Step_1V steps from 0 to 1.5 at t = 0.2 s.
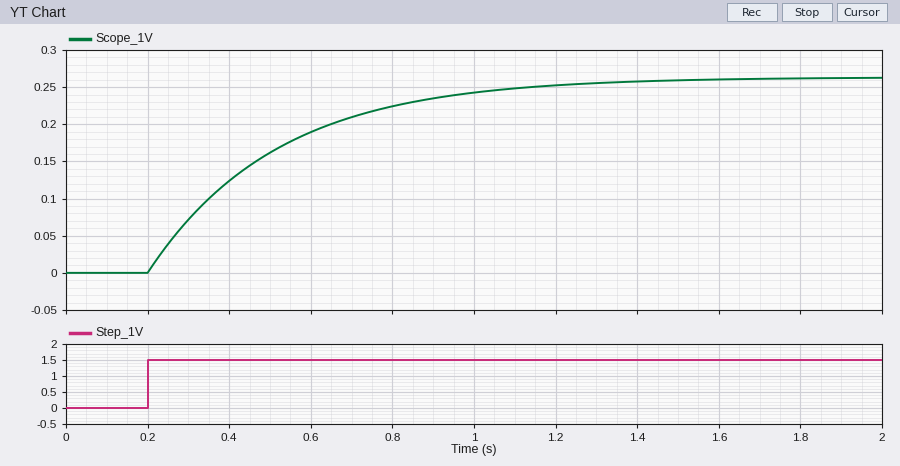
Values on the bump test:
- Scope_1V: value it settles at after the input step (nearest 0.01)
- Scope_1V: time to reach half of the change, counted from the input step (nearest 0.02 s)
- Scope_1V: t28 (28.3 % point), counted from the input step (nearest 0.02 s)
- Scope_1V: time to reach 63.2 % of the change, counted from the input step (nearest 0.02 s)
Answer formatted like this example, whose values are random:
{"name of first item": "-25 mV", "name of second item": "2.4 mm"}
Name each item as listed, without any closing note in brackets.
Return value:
{"Scope_1V: value it settles at after the input step": "0.26", "Scope_1V: time to reach half of the change, counted from the input step": "0.22 s", "Scope_1V: t28 (28.3 % point), counted from the input step": "0.10 s", "Scope_1V: time to reach 63.2 % of the change, counted from the input step": "0.32 s"}
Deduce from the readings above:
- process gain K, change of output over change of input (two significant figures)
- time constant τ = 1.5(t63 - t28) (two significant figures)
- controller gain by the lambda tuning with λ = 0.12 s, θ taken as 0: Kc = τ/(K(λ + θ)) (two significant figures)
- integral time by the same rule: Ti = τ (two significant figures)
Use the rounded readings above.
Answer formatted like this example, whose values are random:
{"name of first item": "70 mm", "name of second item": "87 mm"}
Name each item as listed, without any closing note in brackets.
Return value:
{"process gain K, change of output over change of input": "0.17", "time constant τ = 1.5(t63 - t28)": "0.33 s", "controller gain by the lambda tuning with λ = 0.12 s, θ taken as 0: Kc = τ/(K(λ + θ))": "16", "integral time by the same rule: Ti = τ": "0.33 s"}
